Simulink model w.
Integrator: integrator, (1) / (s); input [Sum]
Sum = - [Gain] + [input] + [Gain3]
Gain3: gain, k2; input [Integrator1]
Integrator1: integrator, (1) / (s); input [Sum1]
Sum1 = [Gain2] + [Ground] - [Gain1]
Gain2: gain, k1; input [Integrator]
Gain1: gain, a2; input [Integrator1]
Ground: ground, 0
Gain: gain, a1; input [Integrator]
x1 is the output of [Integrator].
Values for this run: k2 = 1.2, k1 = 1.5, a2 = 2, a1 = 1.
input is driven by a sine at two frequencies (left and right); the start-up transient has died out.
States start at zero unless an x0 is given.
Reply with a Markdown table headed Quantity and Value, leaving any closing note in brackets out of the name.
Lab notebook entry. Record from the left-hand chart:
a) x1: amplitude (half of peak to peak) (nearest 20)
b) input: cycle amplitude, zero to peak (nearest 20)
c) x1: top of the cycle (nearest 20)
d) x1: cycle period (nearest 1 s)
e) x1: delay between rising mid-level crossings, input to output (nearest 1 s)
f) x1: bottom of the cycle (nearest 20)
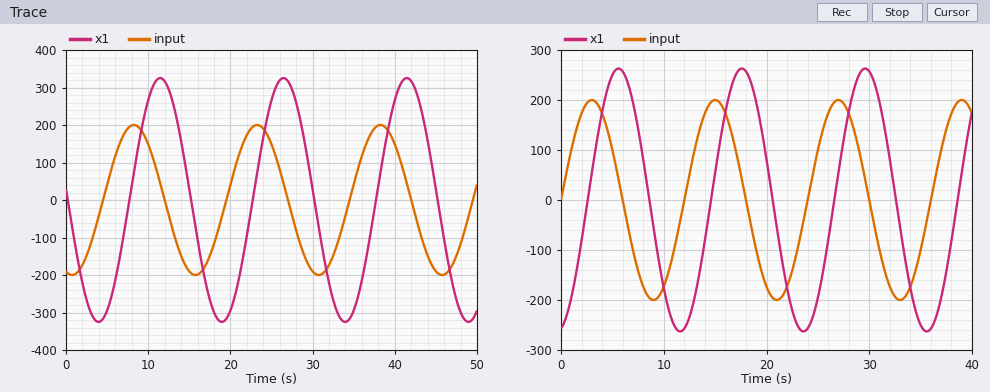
| Quantity | Value |
|---|---|
| x1: amplitude (half of peak to peak) | 320 |
| input: cycle amplitude, zero to peak | 200 |
| x1: top of the cycle | 320 |
| x1: cycle period | 15 s |
| x1: delay between rising mid-level crossings, input to output | 3 s |
| x1: bottom of the cycle | -320 |
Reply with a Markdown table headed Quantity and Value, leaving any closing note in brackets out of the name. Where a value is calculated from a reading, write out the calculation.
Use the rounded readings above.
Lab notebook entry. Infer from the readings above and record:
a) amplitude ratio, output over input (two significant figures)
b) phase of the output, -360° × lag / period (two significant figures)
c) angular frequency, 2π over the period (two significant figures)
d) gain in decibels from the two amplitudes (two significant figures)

| Quantity | Value |
|---|---|
| amplitude ratio, output over input | 320 / 200 = 1.6 |
| phase of the output, -360° × lag / period | -360 × 3 / 15 = -72° |
| angular frequency, 2π over the period | 2π / 15 = 0.42 rad/s |
| gain in decibels from the two amplitudes | 20 log10(320 / 200) = 4.1 dB |
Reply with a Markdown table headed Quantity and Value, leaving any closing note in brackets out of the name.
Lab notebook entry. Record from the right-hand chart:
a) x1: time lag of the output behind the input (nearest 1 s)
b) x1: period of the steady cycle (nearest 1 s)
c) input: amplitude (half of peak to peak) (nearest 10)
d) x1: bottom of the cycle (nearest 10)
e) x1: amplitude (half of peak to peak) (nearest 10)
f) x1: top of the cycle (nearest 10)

| Quantity | Value |
|---|---|
| x1: time lag of the output behind the input | 3 s |
| x1: period of the steady cycle | 12 s |
| input: amplitude (half of peak to peak) | 200 |
| x1: bottom of the cycle | -260 |
| x1: amplitude (half of peak to peak) | 260 |
| x1: top of the cycle | 260 |
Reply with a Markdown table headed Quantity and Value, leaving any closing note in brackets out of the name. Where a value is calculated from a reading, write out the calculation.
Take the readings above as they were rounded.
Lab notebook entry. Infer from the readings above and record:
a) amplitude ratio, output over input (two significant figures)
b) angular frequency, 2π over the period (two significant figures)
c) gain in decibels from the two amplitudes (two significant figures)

| Quantity | Value |
|---|---|
| amplitude ratio, output over input | 260 / 200 = 1.3 |
| angular frequency, 2π over the period | 2π / 12 = 0.52 rad/s |
| gain in decibels from the two amplitudes | 20 log10(260 / 200) = 2.3 dB |
